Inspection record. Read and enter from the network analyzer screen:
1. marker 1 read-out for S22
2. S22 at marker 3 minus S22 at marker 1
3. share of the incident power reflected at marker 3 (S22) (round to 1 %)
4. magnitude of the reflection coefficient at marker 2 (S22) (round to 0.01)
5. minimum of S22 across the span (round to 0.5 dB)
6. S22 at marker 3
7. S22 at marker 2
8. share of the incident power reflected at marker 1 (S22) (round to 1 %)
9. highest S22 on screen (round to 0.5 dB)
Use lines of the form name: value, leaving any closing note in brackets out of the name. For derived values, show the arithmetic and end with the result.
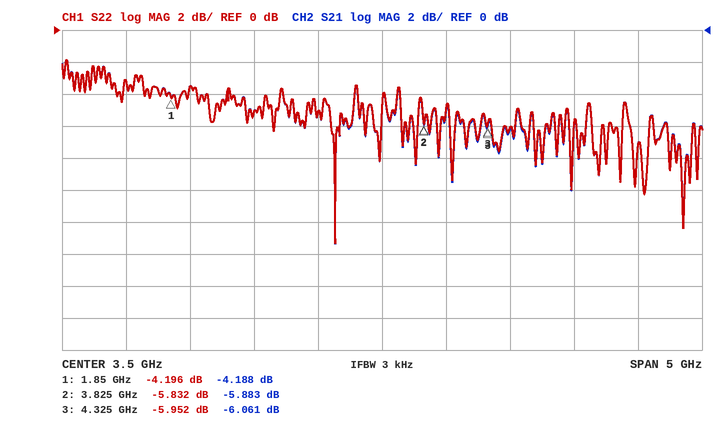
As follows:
marker 1 read-out for S22: -4.196 dB
S22 at marker 3 minus S22 at marker 1: -5.952 − (-4.196) = -1.756 dB
share of the incident power reflected at marker 3 (S22): 10^(-5.952/10) ≈ 25 %
magnitude of the reflection coefficient at marker 2 (S22): 10^(-5.832/20) ≈ 0.51
minimum of S22 across the span: -13.5 dB
S22 at marker 3: -5.952 dB
S22 at marker 2: -5.832 dB
share of the incident power reflected at marker 1 (S22): 10^(-4.196/10) ≈ 38 %
highest S22 on screen: -2.0 dB
